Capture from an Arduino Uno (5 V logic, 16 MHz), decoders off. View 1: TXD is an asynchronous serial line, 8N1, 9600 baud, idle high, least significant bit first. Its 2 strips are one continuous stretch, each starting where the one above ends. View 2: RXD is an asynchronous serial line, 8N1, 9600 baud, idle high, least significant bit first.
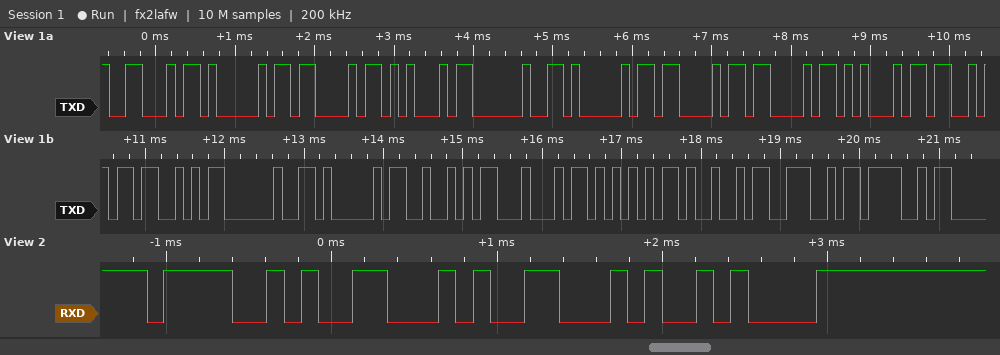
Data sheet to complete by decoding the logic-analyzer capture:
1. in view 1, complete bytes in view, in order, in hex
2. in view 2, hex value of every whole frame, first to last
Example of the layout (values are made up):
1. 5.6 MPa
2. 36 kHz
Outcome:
1. 0x46 0x41 0x43 0x45 0x20 0x41 0x43 0x43 0x45 0x53 0x53 0x20 0x41 0x52 0x44 0x55 0x49 0x4E 0x4F
2. 0x4F 0x46 0x46 0x0A
